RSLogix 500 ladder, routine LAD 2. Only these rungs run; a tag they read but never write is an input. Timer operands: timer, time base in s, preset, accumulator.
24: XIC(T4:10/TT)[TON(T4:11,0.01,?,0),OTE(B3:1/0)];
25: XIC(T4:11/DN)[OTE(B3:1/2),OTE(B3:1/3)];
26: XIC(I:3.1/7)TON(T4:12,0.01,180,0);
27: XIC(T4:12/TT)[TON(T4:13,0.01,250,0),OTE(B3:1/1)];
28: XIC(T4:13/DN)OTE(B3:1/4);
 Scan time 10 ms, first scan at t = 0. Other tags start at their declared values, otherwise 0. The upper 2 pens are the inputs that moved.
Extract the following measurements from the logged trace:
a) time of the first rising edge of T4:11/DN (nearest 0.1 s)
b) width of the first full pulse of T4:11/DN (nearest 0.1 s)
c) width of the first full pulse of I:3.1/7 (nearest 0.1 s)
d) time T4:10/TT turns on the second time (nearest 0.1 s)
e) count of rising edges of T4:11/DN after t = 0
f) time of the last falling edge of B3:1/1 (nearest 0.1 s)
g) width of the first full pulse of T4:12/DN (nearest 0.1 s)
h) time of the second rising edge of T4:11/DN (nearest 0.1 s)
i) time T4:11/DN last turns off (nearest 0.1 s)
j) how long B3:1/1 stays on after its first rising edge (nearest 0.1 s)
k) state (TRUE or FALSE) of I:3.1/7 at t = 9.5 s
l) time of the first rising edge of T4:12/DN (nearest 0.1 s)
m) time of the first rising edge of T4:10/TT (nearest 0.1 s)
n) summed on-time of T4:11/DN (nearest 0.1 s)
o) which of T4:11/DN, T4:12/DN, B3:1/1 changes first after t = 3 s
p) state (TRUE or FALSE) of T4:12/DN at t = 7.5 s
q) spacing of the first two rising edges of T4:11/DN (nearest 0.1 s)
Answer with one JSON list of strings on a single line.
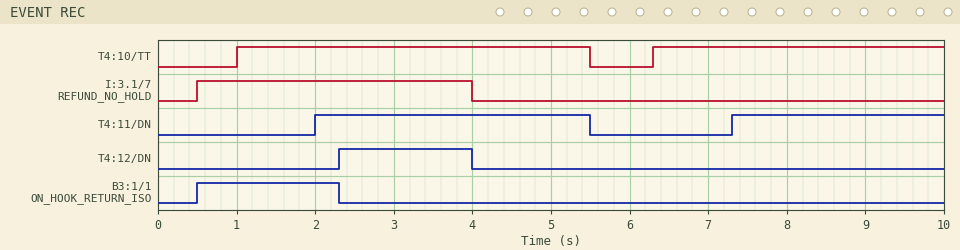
["2.0 s", "3.5 s", "3.5 s", "6.3 s", "2", "2.3 s", "1.7 s", "7.3 s", "5.5 s", "1.8 s", "FALSE", "2.3 s", "1.0 s", "6.2 s", "T4:12/DN", "FALSE", "5.3 s"]
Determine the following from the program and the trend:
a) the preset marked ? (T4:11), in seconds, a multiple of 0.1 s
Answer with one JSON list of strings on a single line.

["1.0 s"]
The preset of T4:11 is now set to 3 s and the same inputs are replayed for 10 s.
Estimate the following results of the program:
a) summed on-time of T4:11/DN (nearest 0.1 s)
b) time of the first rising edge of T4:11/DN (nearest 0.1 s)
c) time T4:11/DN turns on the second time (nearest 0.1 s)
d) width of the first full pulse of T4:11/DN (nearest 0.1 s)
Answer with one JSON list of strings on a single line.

["2.2 s", "4.0 s", "9.3 s", "1.5 s"]
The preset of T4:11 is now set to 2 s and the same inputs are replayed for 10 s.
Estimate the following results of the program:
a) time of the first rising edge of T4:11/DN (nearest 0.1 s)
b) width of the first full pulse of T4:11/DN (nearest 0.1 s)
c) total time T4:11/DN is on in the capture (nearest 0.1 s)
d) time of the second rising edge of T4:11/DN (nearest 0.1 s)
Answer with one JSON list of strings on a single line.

["3.0 s", "2.5 s", "4.2 s", "8.3 s"]
